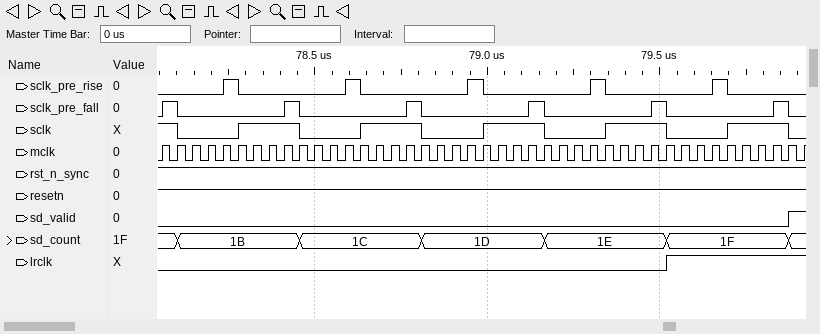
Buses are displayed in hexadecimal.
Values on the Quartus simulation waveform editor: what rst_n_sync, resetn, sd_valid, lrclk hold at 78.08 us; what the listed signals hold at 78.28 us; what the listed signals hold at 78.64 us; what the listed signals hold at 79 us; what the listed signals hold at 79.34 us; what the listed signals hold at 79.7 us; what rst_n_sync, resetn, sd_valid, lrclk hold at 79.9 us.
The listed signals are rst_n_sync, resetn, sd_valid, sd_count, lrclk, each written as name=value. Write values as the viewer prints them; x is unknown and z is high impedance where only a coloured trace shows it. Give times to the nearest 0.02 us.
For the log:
rst_n_sync=1, resetn=1, sd_valid=0, lrclk=0
rst_n_sync=1, resetn=1, sd_valid=0, sd_count=1B, lrclk=0
rst_n_sync=1, resetn=1, sd_valid=0, sd_count=1C, lrclk=0
rst_n_sync=1, resetn=1, sd_valid=0, sd_count=1D, lrclk=0
rst_n_sync=1, resetn=1, sd_valid=0, sd_count=1E, lrclk=0
rst_n_sync=1, resetn=1, sd_valid=0, sd_count=1F, lrclk=1
rst_n_sync=1, resetn=1, sd_valid=1, lrclk=1
